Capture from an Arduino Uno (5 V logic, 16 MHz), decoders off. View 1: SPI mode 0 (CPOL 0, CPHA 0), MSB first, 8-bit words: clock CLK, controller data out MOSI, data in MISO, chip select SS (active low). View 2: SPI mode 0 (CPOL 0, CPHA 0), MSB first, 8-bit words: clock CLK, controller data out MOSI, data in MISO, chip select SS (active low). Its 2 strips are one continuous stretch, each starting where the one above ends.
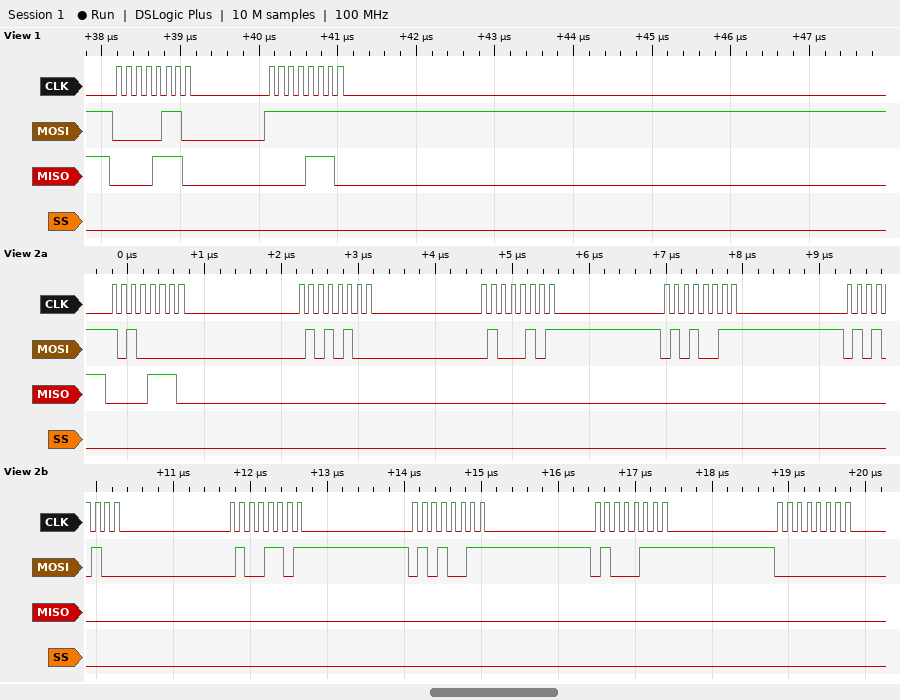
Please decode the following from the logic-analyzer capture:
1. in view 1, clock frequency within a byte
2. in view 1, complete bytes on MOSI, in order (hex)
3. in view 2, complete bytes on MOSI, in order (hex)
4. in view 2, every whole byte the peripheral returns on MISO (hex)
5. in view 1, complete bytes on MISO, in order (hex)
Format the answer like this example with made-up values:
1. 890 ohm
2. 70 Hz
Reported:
1. 8 MHz
2. 06 FF
3. 0xA0 0x54 0x45 0x53 0x54 0x4D 0x53 0x47 0x00
4. 0x0E 0x00 0x00 0x00 0x00 0x00 0x00 0x00 0x00
5. 0E 0E
